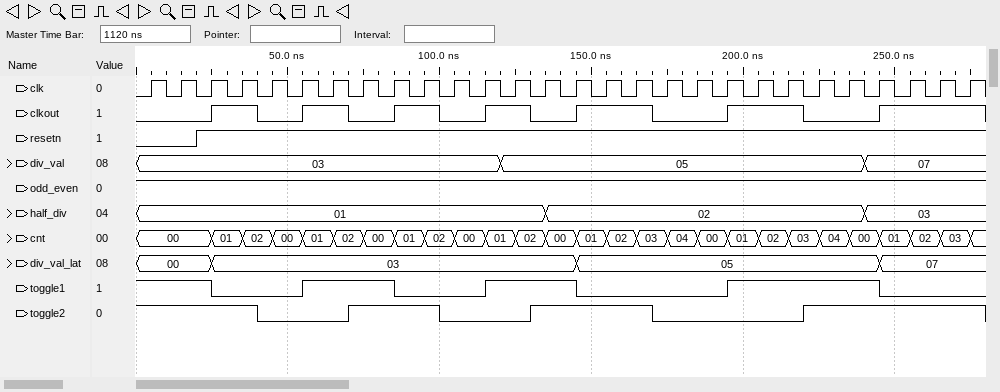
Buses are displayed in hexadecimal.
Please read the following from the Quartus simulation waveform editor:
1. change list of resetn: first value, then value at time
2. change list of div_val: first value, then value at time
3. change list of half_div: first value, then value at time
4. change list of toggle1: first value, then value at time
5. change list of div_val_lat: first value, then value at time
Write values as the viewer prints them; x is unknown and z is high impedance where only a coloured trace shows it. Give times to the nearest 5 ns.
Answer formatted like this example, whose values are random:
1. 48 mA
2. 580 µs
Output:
1. 0, 1 at 20 ns
2. 03, 05 at 120 ns, 07 at 240 ns
3. 01, 02 at 135 ns, 03 at 240 ns
4. 1, 0 at 25 ns, 1 at 55 ns, 0 at 85 ns, 1 at 115 ns, 0 at 145 ns, 1 at 195 ns, 0 at 245 ns
5. 00, 03 at 25 ns, 05 at 145 ns, 07 at 245 ns
